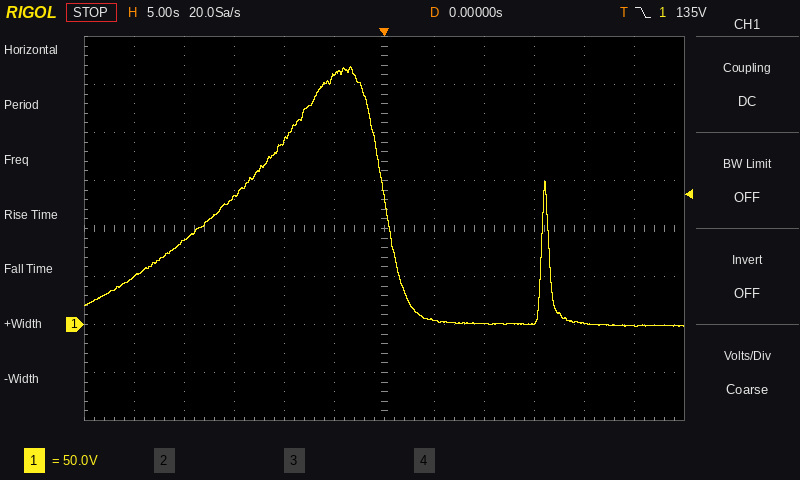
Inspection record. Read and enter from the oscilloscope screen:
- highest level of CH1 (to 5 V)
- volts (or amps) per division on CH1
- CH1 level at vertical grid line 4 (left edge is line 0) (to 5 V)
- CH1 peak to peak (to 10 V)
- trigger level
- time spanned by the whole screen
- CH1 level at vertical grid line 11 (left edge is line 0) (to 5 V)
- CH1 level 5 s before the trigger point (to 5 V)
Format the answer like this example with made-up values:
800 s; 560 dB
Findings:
270 V; 50 V; 190 V; 270 V; 135 V; 60 s; 0 V; 260 V
